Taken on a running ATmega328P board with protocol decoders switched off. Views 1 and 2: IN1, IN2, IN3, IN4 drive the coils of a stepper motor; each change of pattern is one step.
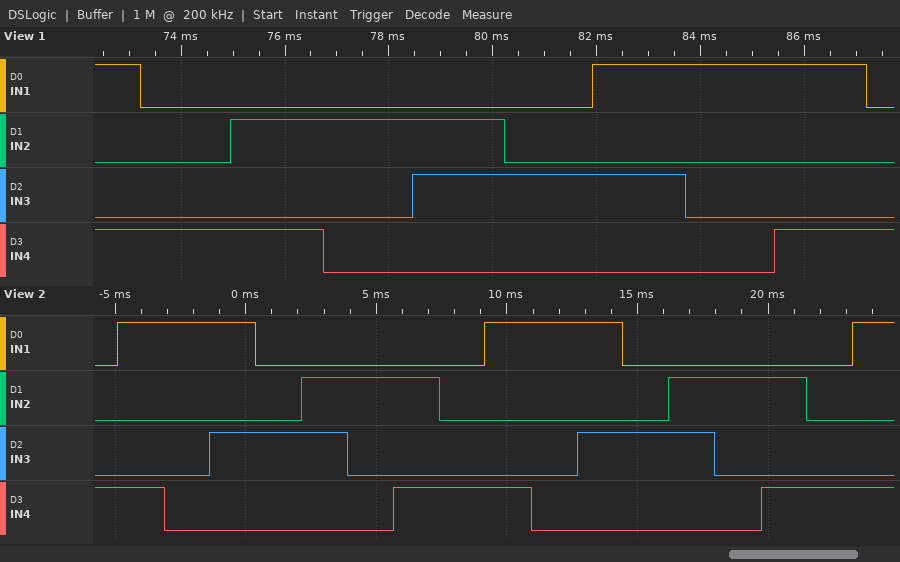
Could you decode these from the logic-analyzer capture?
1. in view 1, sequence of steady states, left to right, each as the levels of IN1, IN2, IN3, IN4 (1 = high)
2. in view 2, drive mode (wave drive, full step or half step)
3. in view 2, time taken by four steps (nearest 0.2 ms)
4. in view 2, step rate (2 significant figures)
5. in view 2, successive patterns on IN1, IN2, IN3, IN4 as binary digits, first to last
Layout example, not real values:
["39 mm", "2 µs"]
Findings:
["1001 0001 0101 0100 0110 0010 1010 1000 1001 0001", "half step", "7.0 ms", "570 steps/s", "0001 1001 1000 1010 0010 0110 0100 0101 0001 1001 1000 1010 0010 0110 0100 0101 0001 1001"]
